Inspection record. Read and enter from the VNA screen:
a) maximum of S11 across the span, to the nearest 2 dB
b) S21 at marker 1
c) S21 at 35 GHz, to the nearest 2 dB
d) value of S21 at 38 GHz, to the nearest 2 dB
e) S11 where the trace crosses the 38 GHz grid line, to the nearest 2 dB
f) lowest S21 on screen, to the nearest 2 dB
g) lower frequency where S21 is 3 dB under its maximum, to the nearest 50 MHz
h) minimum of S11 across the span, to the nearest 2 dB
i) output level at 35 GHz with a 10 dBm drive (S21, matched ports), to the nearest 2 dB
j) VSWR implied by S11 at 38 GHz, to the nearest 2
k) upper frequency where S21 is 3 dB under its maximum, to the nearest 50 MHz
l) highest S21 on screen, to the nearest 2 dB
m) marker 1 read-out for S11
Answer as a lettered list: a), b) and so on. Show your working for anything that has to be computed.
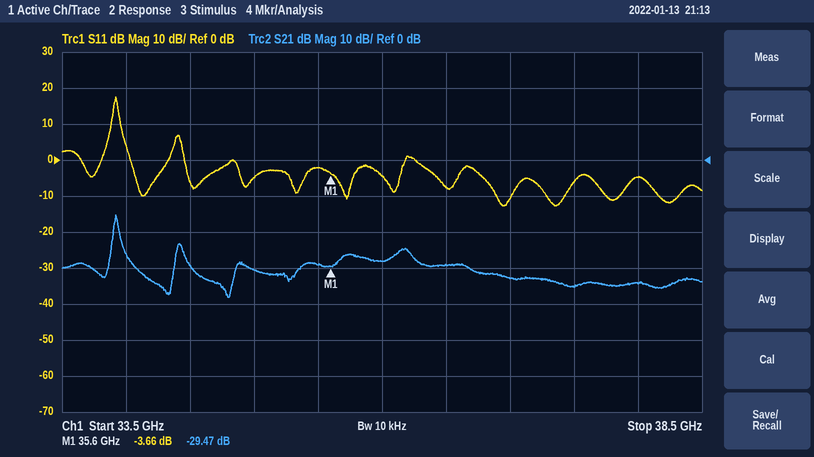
a) 18 dB
b) -29.47 dB
c) -30 dB
d) -34 dB
e) -4 dB
f) -38 dB
g) 33.90 GHz
h) -12 dB
i) 10 dBm + (-30 dB) = -20 dBm
j) |Γ| = 10^(-4/20) = 0.6310; VSWR = (1 + 0.6310)/(1 − 0.6310) ≈ 4
k) 33.95 GHz
l) -16 dB
m) -3.66 dB
